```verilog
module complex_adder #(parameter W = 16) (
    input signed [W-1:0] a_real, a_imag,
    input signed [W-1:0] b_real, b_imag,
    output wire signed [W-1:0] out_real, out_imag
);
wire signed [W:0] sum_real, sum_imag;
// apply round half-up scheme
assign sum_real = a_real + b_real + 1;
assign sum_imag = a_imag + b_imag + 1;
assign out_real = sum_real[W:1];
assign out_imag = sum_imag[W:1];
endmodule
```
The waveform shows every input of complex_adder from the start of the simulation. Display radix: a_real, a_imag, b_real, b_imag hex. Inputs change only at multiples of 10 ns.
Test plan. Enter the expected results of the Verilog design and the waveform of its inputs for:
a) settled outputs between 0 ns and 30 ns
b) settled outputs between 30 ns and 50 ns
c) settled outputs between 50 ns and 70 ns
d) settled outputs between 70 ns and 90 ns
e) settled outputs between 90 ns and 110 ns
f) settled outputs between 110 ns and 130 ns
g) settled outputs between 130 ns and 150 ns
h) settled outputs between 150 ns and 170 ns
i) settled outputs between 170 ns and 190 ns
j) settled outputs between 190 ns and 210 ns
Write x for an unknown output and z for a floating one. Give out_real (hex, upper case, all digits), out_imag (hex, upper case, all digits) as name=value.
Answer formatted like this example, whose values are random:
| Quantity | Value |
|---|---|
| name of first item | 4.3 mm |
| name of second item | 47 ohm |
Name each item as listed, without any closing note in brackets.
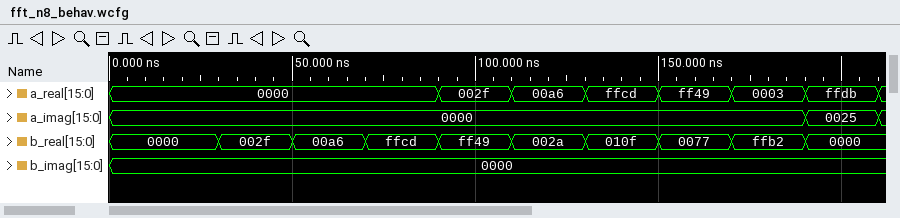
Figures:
| Quantity | Value |
|---|---|
| settled outputs between 0 ns and 30 ns | out_real=0000, out_imag=0000 |
| settled outputs between 30 ns and 50 ns | out_real=0018, out_imag=0000 |
| settled outputs between 50 ns and 70 ns | out_real=0053, out_imag=0000 |
| settled outputs between 70 ns and 90 ns | out_real=FFE7, out_imag=0000 |
| settled outputs between 90 ns and 110 ns | out_real=FFBC, out_imag=0000 |
| settled outputs between 110 ns and 130 ns | out_real=0068, out_imag=0000 |
| settled outputs between 130 ns and 150 ns | out_real=006E, out_imag=0000 |
| settled outputs between 150 ns and 170 ns | out_real=FFE0, out_imag=0000 |
| settled outputs between 170 ns and 190 ns | out_real=FFDB, out_imag=0000 |
| settled outputs between 190 ns and 210 ns | out_real=FFEE, out_imag=0013 |
